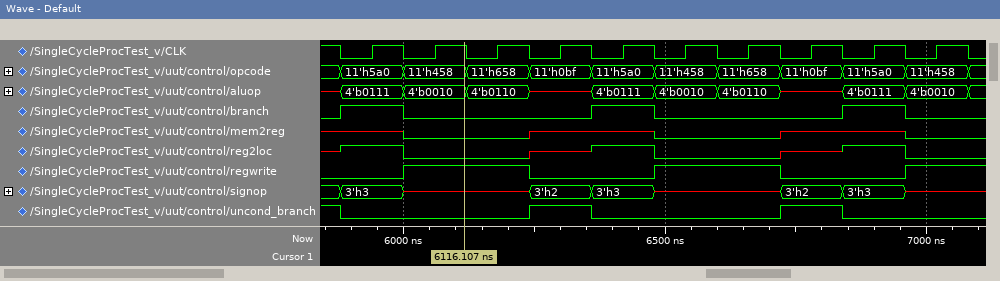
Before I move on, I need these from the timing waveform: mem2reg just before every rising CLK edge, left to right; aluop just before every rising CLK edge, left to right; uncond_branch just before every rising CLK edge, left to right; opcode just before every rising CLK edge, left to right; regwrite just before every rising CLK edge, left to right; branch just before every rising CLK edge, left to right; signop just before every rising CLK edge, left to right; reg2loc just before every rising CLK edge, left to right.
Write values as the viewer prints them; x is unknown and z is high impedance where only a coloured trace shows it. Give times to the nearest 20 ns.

x 0 0 x x 0 0 x x 0
4'b0111, 4'b0010, 4'b0110, x, 4'b0111, 4'b0010, 4'b0110, x, 4'b0111, 4'b0010
0 0 0 1 0 0 0 1 0 0
11'h5a0, 11'h458, 11'h658, 11'h0bf, 11'h5a0, 11'h458, 11'h658, 11'h0bf, 11'h5a0, 11'h458
0 1 1 0 0 1 1 0 0 1
1 0 0 0 1 0 0 0 1 0
3'h3, x, x, 3'h2, 3'h3, x, x, 3'h2, 3'h3, x
1 0 0 x 1 0 0 x 1 0
